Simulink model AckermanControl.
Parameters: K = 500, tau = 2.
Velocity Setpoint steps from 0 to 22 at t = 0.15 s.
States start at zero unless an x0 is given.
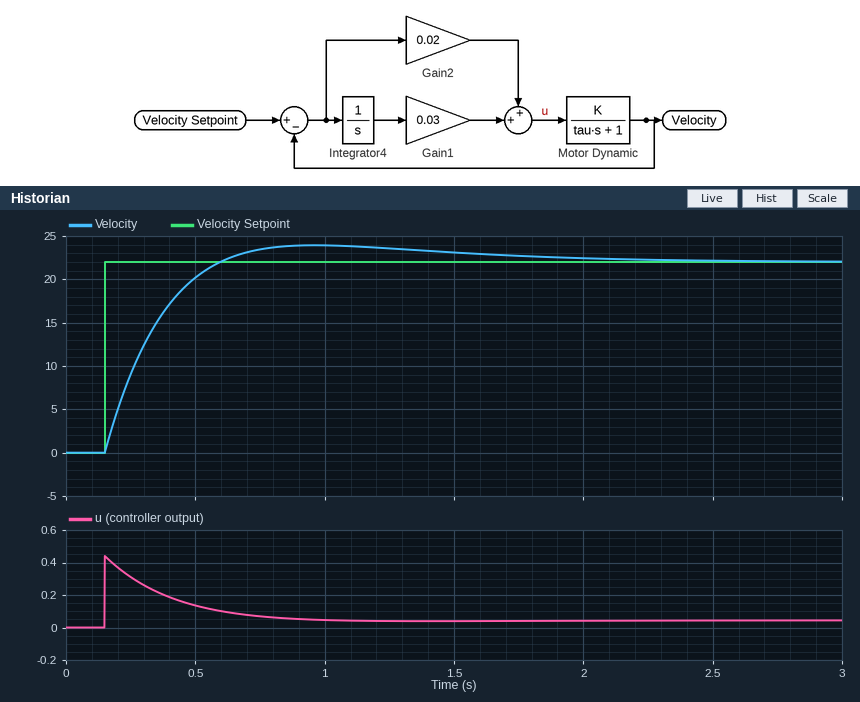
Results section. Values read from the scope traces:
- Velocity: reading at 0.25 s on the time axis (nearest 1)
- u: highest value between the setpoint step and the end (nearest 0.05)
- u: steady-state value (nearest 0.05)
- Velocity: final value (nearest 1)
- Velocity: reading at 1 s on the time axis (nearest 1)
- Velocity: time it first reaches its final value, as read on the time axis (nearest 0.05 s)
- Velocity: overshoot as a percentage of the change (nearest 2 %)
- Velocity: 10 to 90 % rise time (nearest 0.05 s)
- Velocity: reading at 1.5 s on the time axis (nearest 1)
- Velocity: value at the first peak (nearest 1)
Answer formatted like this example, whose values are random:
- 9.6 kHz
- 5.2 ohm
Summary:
- 9
- 0.45
- 0.05
- 22
- 24
- 0.60 s
- 8 %
- 0.30 s
- 23
- 24
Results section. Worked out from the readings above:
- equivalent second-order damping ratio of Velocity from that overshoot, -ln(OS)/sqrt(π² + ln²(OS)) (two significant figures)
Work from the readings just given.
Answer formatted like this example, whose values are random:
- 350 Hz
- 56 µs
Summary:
- 0.63
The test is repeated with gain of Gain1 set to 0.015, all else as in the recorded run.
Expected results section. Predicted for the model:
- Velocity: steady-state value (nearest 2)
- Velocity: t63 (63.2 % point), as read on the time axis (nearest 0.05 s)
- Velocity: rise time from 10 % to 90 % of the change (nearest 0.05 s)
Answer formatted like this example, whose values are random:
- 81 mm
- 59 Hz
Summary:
- 22
- 0.35 s
- 0.40 s
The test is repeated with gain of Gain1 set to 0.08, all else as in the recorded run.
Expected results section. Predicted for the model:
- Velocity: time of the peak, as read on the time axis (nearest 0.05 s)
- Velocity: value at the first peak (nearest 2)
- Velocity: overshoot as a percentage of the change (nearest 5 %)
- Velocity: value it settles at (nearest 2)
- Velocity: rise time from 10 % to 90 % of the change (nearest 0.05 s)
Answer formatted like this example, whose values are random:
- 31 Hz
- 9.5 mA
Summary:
- 0.70 s
- 26
- 20 %
- 22
- 0.20 s
